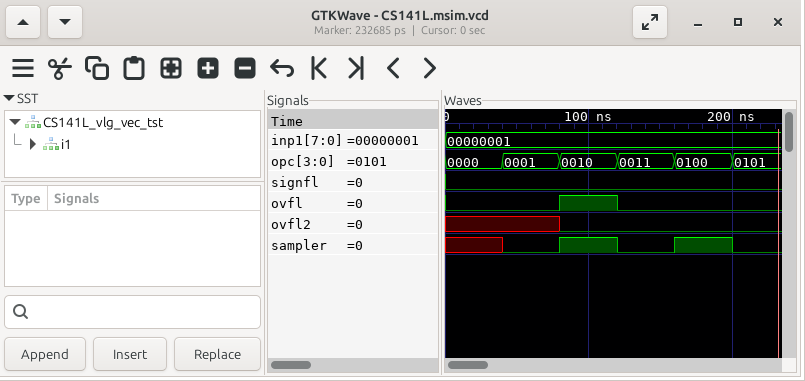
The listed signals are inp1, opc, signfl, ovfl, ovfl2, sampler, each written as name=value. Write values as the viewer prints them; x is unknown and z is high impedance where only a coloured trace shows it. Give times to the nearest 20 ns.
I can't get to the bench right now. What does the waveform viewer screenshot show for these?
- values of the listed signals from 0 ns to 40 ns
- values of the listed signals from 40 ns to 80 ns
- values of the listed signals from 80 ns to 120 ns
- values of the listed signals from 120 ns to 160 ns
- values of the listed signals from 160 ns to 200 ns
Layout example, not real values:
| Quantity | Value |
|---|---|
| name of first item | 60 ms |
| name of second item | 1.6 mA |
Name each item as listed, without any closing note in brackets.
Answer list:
| Quantity | Value |
|---|---|
| values of the listed signals from 0 ns to 40 ns | inp1=00000001, opc=0000, signfl=0, ovfl=0, ovfl2=x, sampler=x |
| values of the listed signals from 40 ns to 80 ns | inp1=00000001, opc=0001, signfl=0, ovfl=0, ovfl2=x, sampler=0 |
| values of the listed signals from 80 ns to 120 ns | inp1=00000001, opc=0010, signfl=0, ovfl=1, ovfl2=0, sampler=1 |
| values of the listed signals from 120 ns to 160 ns | inp1=00000001, opc=0011, signfl=0, ovfl=0, ovfl2=0, sampler=0 |
| values of the listed signals from 160 ns to 200 ns | inp1=00000001, opc=0100, signfl=0, ovfl=0, ovfl2=0, sampler=1 |
